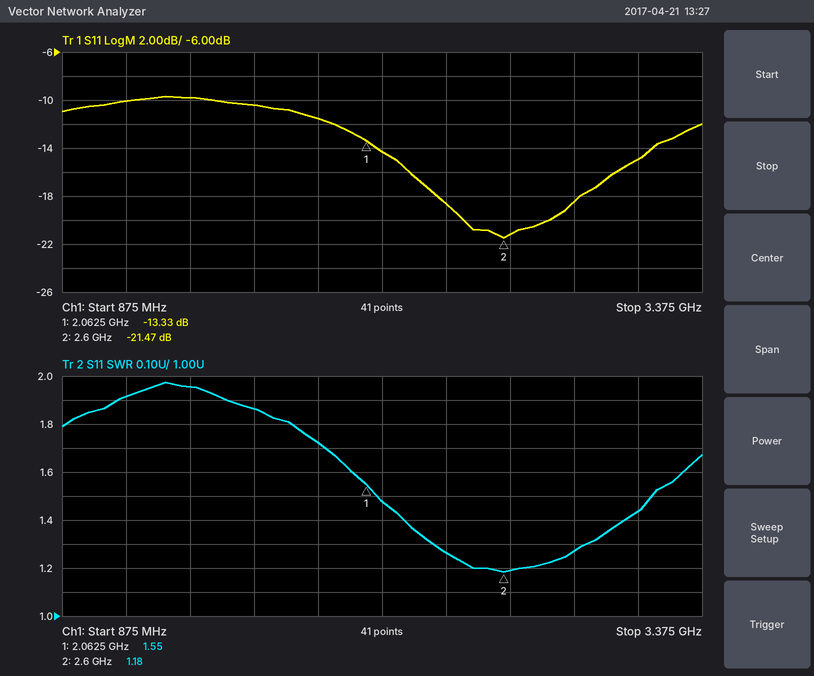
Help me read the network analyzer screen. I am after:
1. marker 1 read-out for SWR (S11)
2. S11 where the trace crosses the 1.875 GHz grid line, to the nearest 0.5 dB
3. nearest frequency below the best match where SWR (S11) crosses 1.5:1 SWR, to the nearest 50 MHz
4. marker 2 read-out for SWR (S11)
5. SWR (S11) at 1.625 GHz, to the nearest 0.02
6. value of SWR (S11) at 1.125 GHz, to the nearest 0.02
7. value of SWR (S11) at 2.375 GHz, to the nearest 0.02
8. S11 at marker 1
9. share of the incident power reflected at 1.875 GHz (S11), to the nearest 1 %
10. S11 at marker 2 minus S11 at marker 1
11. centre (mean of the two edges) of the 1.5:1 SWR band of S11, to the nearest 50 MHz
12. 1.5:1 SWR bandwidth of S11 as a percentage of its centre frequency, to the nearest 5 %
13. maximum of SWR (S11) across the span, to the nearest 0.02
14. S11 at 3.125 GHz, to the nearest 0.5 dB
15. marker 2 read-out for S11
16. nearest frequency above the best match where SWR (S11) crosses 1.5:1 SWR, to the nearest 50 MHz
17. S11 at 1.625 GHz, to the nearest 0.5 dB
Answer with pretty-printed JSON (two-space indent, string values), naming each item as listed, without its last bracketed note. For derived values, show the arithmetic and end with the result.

{
  "marker 1 read-out for SWR": "1.55",
  "S11 where the trace crosses the 1.875 GHz grid line, to the nearest 0.5 dB": "-11.5 dB",
  "nearest frequency below the best match where SWR (S11) crosses 1.5:1 SWR, to the nearest 50 MHz": "2.10 GHz",
  "marker 2 read-out for SWR": "1.18",
  "SWR (S11) at 1.625 GHz, to the nearest 0.02": "1.86",
  "value of SWR (S11) at 1.125 GHz, to the nearest 0.02": "1.92",
  "value of SWR (S11) at 2.375 GHz, to the nearest 0.02": "1.26",
  "S11 at marker 1": "-13.33 dB",
  "share of the incident power reflected at 1.875 GHz (S11), to the nearest 1 %": "10^(-11.5/10) ≈ 7 %",
  "S11 at marker 2 minus S11 at marker 1": "-21.47 − (-13.33) = -8.14 dB",
  "centre (mean of the two edges) of the 1.5:1 SWR band of S11, to the nearest 50 MHz": "2.65 GHz",
  "1.5:1 SWR bandwidth of S11 as a percentage of its centre frequency, to the nearest 5 %": "1.1 GHz / 2.65 GHz ≈ 41.5 %, so 40 % to the nearest 5 %",
  "maximum of SWR (S11) across the span, to the nearest 0.02": "1.98",
  "S11 at 3.125 GHz, to the nearest 0.5 dB": "-15.0 dB",
  "marker 2 read-out for S11": "-21.47 dB",
  "nearest frequency above the best match where SWR (S11) crosses 1.5:1 SWR, to the nearest 50 MHz": "3.20 GHz",
  "S11 at 1.625 GHz, to the nearest 0.5 dB": "-10.5 dB"
}
